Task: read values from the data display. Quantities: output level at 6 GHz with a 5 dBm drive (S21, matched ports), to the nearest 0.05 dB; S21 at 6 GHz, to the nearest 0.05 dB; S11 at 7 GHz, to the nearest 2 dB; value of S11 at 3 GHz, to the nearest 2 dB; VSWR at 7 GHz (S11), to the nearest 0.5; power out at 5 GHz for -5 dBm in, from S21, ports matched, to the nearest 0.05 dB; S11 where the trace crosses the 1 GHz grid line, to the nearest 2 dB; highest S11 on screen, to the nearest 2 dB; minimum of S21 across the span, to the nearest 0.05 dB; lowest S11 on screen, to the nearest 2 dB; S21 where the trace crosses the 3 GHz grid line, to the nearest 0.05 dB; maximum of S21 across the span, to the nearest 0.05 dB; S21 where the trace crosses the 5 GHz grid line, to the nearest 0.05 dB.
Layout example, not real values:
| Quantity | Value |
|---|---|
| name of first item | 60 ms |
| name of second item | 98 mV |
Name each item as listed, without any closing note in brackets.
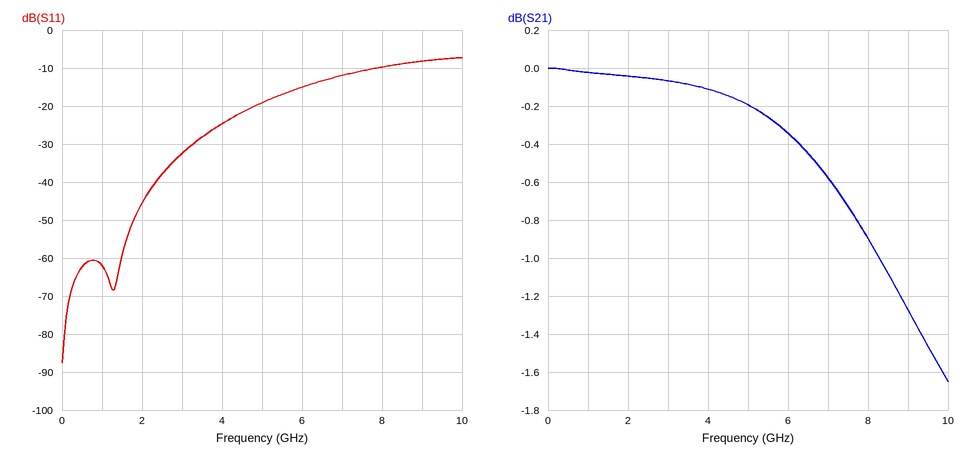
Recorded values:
| Quantity | Value |
|---|---|
| output level at 6 GHz with a 5 dBm drive (S21, matched ports), to the nearest 0.05 dB | 4.65 dBm |
| S21 at 6 GHz, to the nearest 0.05 dB | -0.35 dB |
| S11 at 7 GHz, to the nearest 2 dB | -12 dB |
| value of S11 at 3 GHz, to the nearest 2 dB | -32 dB |
| VSWR at 7 GHz (S11), to the nearest 0.5 | 1.5 |
| power out at 5 GHz for -5 dBm in, from S21, ports matched, to the nearest 0.05 dB | -5.20 dBm |
| S11 where the trace crosses the 1 GHz grid line, to the nearest 2 dB | -62 dB |
| highest S11 on screen, to the nearest 2 dB | -8 dB |
| minimum of S21 across the span, to the nearest 0.05 dB | -1.65 dB |
| lowest S11 on screen, to the nearest 2 dB | -88 dB |
| S21 where the trace crosses the 3 GHz grid line, to the nearest 0.05 dB | -0.05 dB |
| maximum of S21 across the span, to the nearest 0.05 dB | 0.00 dB |
| S21 where the trace crosses the 5 GHz grid line, to the nearest 0.05 dB | -0.20 dB |
